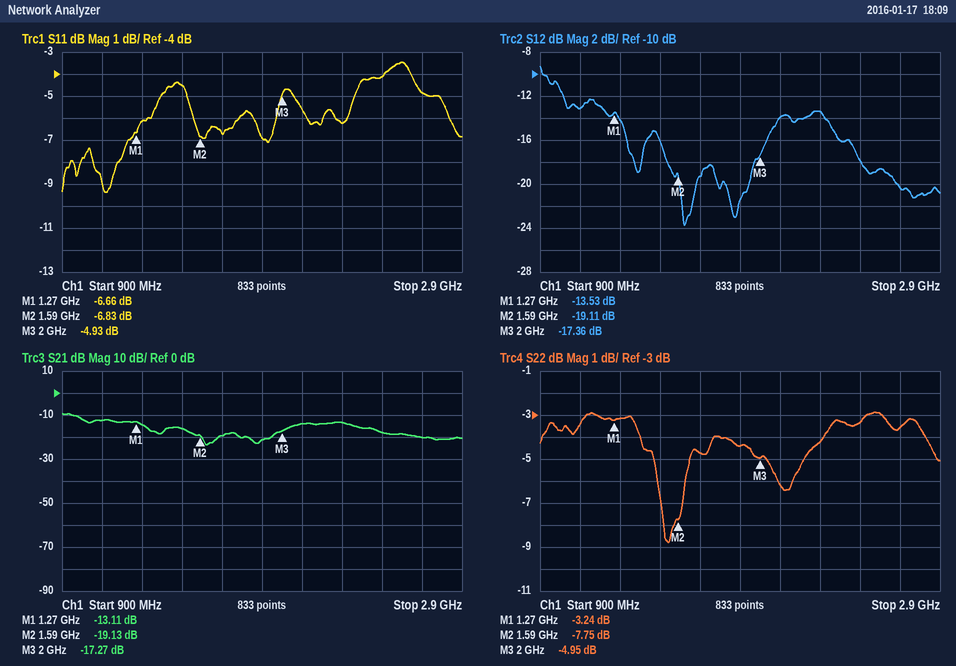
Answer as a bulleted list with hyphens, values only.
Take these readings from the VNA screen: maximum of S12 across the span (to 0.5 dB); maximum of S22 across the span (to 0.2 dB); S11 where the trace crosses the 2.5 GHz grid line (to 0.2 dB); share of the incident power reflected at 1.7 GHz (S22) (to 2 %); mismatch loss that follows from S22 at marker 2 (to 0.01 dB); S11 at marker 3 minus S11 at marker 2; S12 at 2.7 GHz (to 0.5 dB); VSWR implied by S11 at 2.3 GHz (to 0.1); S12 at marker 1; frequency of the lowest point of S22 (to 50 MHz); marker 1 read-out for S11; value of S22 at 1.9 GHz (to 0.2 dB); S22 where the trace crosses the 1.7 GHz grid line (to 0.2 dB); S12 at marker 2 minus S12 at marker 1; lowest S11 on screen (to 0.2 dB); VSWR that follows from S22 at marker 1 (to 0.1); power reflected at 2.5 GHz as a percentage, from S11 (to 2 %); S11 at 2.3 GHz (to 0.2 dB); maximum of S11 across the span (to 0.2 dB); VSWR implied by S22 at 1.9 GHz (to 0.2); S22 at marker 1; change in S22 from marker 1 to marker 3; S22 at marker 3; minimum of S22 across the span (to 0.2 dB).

- -9.5 dB
- -2.8 dB
- -4.2 dB
- 34 %
- 0.80 dB
- 1.90 dB
- -20.5 dB
- 2.9
- -13.53 dB
- 1.55 GHz
- -6.66 dB
- -4.4 dB
- -4.8 dB
- -5.58 dB
- -9.4 dB
- 5.4
- 38 %
- -6.2 dB
- -3.4 dB
- 4.0
- -3.24 dB
- -1.71 dB
- -4.95 dB
- -8.8 dB
